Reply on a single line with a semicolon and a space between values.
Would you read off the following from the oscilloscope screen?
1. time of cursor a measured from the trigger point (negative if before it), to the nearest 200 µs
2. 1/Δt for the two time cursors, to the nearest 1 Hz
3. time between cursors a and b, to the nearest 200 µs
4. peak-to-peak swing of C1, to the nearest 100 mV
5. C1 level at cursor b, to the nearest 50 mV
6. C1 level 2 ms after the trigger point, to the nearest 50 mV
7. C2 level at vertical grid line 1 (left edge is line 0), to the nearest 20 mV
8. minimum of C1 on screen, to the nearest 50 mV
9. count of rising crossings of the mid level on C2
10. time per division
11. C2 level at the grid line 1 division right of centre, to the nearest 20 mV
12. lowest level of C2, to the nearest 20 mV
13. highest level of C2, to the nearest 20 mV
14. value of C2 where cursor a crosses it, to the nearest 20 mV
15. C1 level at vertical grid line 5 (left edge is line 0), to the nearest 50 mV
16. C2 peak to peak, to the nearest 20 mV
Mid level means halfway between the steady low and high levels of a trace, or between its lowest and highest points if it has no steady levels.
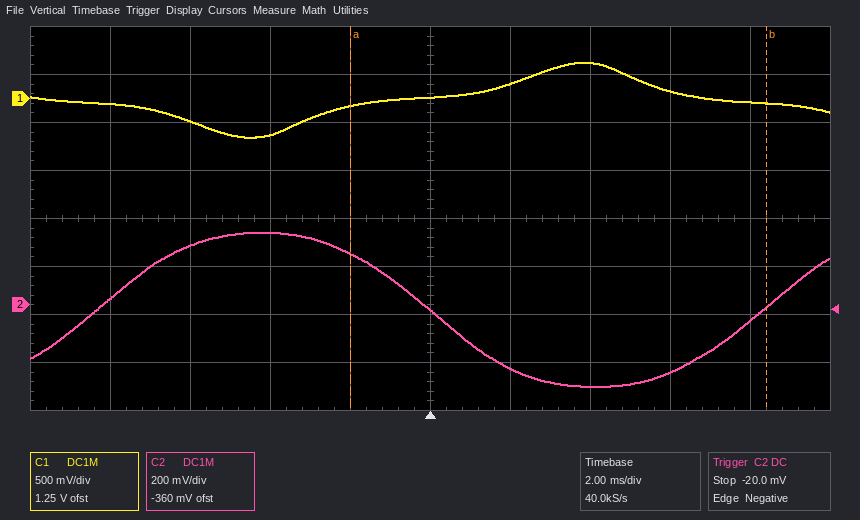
-2.0 ms; 96 Hz; 10.4 ms; 800 mV; -50 mV; 150 mV; 20 mV; -400 mV; 2; 2 ms; -260 mV; -340 mV; 300 mV; 220 mV; 0 mV; 640 mV
